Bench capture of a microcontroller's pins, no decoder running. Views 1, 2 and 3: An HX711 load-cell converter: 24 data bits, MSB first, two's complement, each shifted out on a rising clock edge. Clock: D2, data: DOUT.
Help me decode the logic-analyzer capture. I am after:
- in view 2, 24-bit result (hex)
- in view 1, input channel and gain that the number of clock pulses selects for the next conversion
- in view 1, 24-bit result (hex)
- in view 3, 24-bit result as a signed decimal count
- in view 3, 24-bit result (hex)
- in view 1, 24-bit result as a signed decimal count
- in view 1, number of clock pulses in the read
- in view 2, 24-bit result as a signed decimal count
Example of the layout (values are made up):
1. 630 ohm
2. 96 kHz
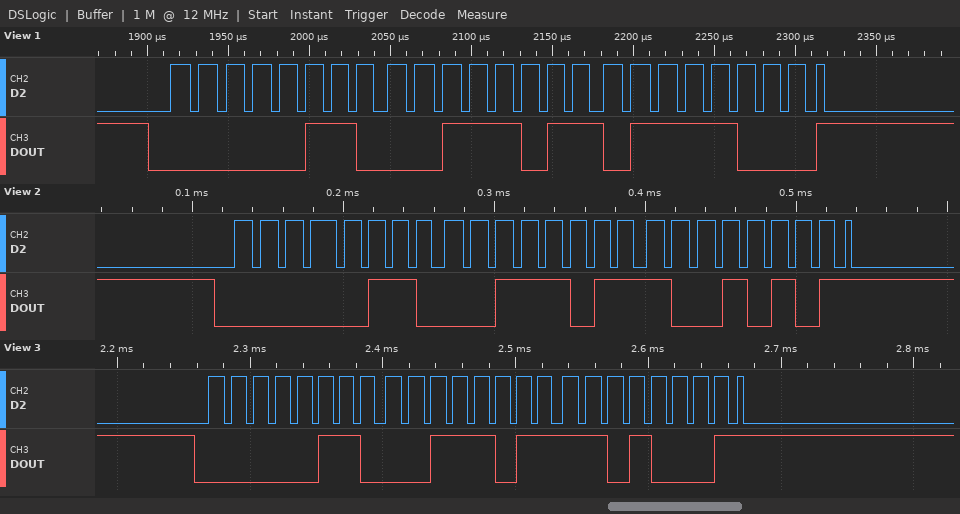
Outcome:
1. 0x063B95
2. channel A, gain 128
3. 0x063B78
4. 408529
5. 0x063BD1
6. 408440
7. 25
8. 408469
